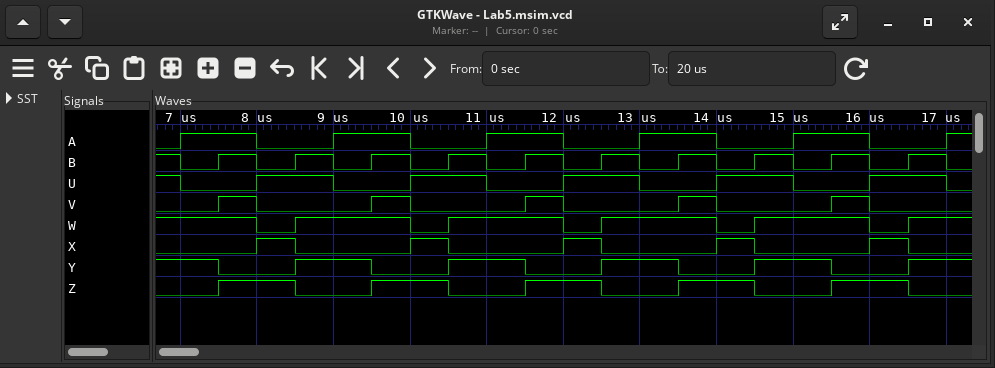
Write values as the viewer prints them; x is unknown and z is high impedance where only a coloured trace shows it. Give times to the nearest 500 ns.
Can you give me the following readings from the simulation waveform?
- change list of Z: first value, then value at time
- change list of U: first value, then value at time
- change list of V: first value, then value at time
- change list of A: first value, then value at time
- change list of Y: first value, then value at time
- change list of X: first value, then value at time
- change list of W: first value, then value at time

0, 1 at 7500 ns, 0 at 8500 ns, 1 at 9500 ns, 0 at 10500 ns, 1 at 11500 ns, 0 at 12500 ns, 1 at 13500 ns, 0 at 14500 ns, 1 at 15500 ns, 0 at 16500 ns
1, 0 at 7000 ns, 1 at 8000 ns, 0 at 9000 ns, 1 at 10000 ns, 0 at 11000 ns, 1 at 12000 ns, 0 at 13000 ns, 1 at 14000 ns, 0 at 15000 ns, 1 at 16000 ns, 0 at 17000 ns
0, 1 at 7500 ns, 0 at 8000 ns, 1 at 9500 ns, 0 at 10000 ns, 1 at 11500 ns, 0 at 12000 ns, 1 at 13500 ns, 0 at 14000 ns, 1 at 15500 ns, 0 at 16000 ns
0, 1 at 7000 ns, 0 at 8000 ns, 1 at 9000 ns, 0 at 10000 ns, 1 at 11000 ns, 0 at 12000 ns, 1 at 13000 ns, 0 at 14000 ns, 1 at 15000 ns, 0 at 16000 ns, 1 at 17000 ns
1, 0 at 7500 ns, 1 at 8500 ns, 0 at 9500 ns, 1 at 10500 ns, 0 at 11500 ns, 1 at 12500 ns, 0 at 13500 ns, 1 at 14500 ns, 0 at 15500 ns, 1 at 16500 ns
0, 1 at 8000 ns, 0 at 8500 ns, 1 at 10000 ns, 0 at 10500 ns, 1 at 12000 ns, 0 at 12500 ns, 1 at 14000 ns, 0 at 14500 ns, 1 at 16000 ns, 0 at 16500 ns
1, 0 at 8000 ns, 1 at 8500 ns, 0 at 10000 ns, 1 at 10500 ns, 0 at 12000 ns, 1 at 12500 ns, 0 at 14000 ns, 1 at 14500 ns, 0 at 16000 ns, 1 at 16500 ns
